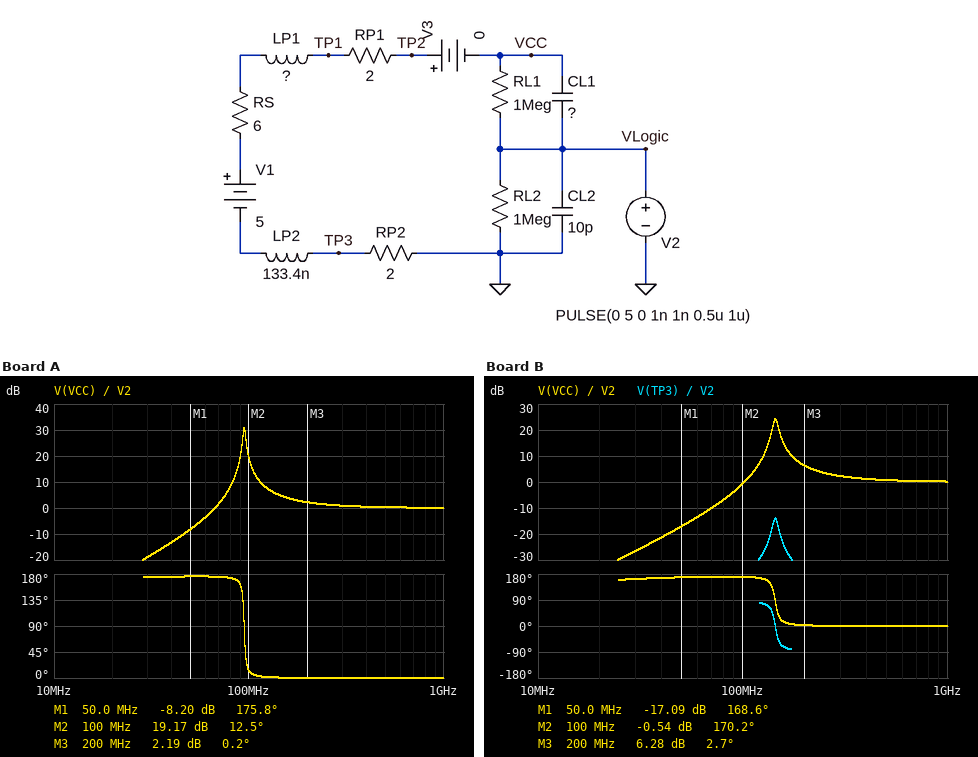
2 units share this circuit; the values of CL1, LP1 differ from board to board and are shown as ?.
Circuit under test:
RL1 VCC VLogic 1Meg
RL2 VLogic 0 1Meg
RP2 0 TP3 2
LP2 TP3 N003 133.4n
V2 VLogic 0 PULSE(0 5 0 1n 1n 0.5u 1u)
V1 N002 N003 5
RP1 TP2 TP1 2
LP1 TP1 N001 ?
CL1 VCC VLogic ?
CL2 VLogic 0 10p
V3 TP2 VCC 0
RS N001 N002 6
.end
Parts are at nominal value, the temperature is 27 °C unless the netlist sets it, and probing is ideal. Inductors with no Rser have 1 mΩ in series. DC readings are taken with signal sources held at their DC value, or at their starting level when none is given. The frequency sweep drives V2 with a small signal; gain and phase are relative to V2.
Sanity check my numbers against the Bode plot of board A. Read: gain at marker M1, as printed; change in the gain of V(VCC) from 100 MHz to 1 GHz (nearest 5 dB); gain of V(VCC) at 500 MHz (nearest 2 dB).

-8.20 dB
-20 dB
0 dB
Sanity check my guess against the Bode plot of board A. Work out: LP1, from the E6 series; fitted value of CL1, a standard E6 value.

470 nH
4.7 pF
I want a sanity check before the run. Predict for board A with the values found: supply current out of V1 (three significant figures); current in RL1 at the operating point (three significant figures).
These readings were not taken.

5.00 µA
5.00 µA
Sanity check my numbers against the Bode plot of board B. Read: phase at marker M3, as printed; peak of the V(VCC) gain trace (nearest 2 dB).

2.7 deg
24 dB
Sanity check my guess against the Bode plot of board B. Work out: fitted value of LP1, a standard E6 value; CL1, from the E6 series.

47 nH
6.8 pF
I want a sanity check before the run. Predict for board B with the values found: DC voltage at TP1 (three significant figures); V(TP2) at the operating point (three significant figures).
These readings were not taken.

5.00 V
5.00 V
